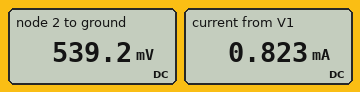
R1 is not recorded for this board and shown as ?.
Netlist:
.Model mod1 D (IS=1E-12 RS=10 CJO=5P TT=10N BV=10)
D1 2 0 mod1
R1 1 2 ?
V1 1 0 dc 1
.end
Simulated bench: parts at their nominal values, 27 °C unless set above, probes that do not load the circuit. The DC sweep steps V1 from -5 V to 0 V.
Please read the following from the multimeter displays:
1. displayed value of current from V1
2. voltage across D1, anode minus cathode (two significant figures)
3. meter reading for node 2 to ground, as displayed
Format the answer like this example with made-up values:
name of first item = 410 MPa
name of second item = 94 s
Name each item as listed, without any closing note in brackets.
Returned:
displayed value of current from V1 = 0.823 mA
voltage across D1, anode minus cathode = 540 mV
meter reading for node 2 to ground, as displayed = 539.2 mV
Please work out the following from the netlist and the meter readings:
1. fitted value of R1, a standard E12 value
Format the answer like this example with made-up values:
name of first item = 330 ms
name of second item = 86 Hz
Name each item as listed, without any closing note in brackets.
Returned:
fitted value of R1, a standard E12 value = 560 Ω
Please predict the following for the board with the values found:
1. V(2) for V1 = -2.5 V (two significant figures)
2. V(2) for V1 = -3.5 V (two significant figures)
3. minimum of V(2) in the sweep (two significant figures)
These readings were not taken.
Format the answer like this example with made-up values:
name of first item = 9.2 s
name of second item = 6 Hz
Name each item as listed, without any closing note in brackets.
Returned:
V(2) for V1 = -2.5 V = -2.5 V
V(2) for V1 = -3.5 V = -3.5 V
minimum of V(2) in the sweep = -5.0 V
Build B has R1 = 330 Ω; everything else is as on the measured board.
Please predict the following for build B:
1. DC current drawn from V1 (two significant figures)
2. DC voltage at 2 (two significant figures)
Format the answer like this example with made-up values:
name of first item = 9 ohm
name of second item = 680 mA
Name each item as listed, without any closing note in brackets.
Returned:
DC current drawn from V1 = 1.3 mA
DC voltage at 2 = 560 mV
